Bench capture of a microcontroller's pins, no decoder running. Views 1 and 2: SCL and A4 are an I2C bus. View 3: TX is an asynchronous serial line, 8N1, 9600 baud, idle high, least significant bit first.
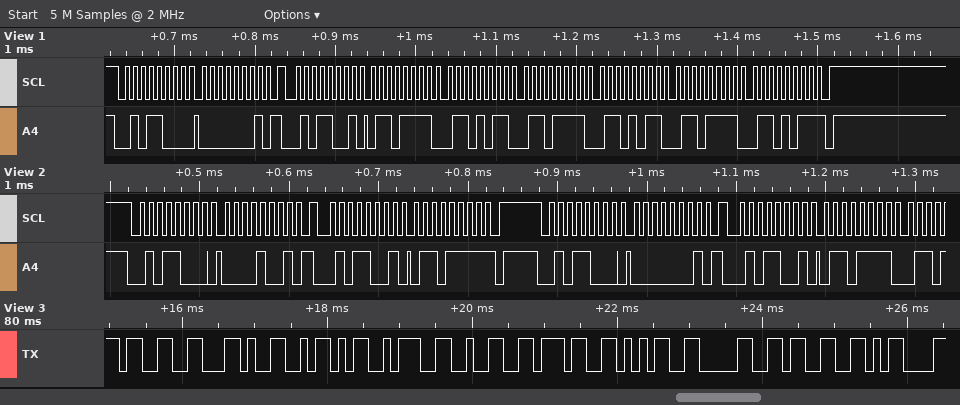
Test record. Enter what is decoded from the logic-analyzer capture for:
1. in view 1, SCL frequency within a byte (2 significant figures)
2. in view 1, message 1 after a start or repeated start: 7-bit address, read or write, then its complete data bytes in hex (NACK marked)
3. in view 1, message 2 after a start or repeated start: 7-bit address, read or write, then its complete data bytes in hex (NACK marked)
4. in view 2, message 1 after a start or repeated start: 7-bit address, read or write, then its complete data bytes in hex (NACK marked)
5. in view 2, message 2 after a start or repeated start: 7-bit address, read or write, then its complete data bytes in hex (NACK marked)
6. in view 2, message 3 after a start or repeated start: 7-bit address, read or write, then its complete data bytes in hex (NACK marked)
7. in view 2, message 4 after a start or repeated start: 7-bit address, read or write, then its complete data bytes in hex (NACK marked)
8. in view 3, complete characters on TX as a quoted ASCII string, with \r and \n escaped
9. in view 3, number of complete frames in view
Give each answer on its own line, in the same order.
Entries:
100 kHz
0x2C write: 01
0x2C read: 6F 6B 6F 6B 6F 6B NACK
0x2C write: 09
0x2C read: 6F NACK
0x2C write: 01
0x2C read: 6F
"3,Z:27503\r"
10
